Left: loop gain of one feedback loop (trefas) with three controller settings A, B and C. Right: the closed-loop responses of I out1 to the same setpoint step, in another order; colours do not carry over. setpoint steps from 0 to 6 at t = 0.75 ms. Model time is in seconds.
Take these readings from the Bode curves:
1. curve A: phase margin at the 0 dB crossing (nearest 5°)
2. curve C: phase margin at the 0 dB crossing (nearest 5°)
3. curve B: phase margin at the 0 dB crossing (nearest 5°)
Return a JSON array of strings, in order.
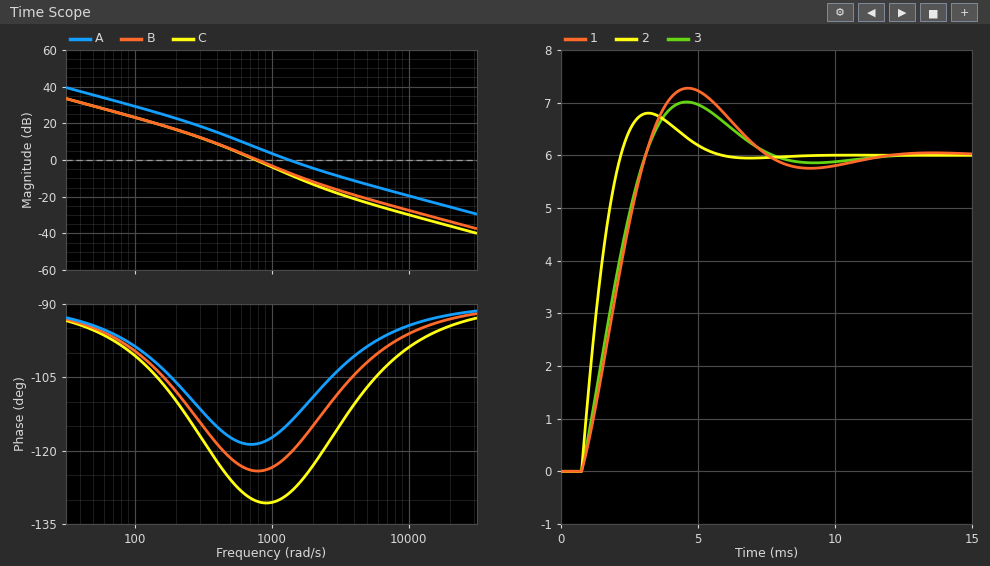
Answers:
["65°", "50°", "55°"]
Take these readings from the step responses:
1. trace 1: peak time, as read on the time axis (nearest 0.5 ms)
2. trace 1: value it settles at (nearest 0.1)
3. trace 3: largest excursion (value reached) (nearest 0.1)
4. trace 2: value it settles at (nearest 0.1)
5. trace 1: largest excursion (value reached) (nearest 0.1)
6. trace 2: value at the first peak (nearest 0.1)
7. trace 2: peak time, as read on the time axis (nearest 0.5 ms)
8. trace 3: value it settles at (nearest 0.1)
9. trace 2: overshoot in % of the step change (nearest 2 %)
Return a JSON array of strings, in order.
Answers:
["4.5 ms", "6.0", "7.0", "6.0", "7.3", "6.8", "3.0 ms", "6.0", "14 %"]
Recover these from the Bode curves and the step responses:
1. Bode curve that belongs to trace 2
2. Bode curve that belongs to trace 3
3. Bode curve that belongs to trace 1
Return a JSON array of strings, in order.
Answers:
["A", "B", "C"]
